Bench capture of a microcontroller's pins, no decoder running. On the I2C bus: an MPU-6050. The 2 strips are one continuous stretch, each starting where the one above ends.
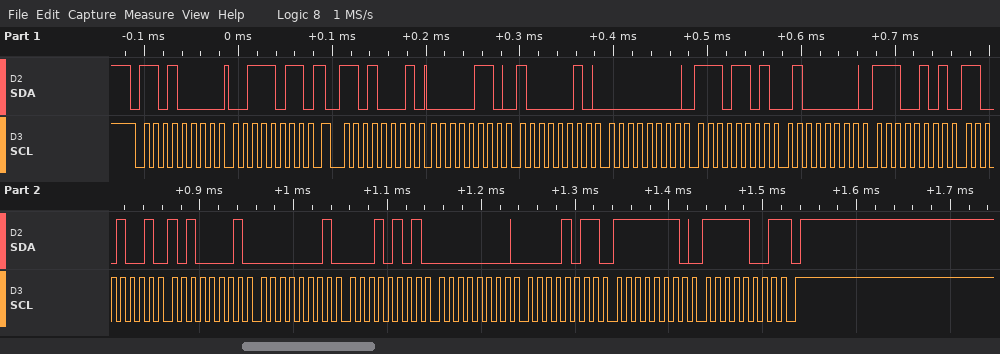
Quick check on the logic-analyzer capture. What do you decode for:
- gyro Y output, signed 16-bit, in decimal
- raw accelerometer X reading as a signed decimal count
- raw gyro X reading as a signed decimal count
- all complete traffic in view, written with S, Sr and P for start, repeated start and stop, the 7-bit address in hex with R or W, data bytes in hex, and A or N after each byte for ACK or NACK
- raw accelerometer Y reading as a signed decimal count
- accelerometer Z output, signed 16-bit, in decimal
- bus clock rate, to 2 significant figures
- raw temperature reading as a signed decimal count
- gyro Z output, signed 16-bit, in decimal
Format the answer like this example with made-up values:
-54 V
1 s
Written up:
11
1666
277
S 68W A 3B A Sr 68R A 06 A 82 A 00 A ED A 40 A E5 A C9 A A1 A 01 A 15 A 00 A 0B A FE A F9 N P
237
16613
100 kHz
-13919
-263
